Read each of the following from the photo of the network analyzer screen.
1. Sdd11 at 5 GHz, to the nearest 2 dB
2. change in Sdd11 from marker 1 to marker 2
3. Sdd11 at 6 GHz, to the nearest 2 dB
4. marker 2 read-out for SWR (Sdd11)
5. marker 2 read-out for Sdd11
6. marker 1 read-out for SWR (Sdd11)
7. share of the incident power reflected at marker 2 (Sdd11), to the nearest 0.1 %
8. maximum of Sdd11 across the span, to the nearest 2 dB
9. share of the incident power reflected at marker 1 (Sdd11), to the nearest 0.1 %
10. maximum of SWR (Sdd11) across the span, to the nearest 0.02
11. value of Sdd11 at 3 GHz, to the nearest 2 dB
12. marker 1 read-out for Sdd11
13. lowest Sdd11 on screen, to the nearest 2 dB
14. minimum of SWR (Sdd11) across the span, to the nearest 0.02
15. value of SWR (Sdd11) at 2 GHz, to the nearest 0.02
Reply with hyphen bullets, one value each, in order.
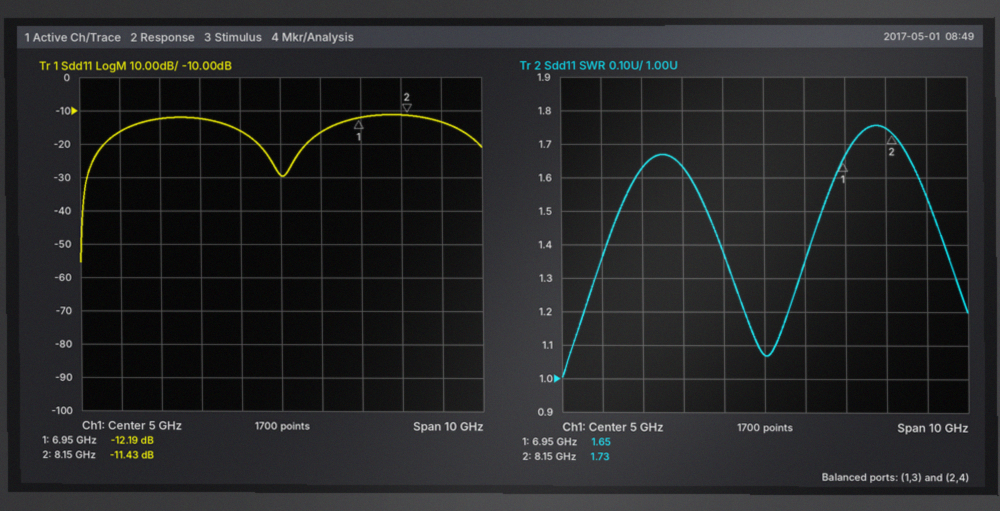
- -30 dB
- 0.76 dB
- -16 dB
- 1.73
- -11.43 dB
- 1.65
- 7.2 %
- -12 dB
- 6.0 %
- 1.76
- -12 dB
- -12.19 dB
- -56 dB
- 1.00
- 1.62
